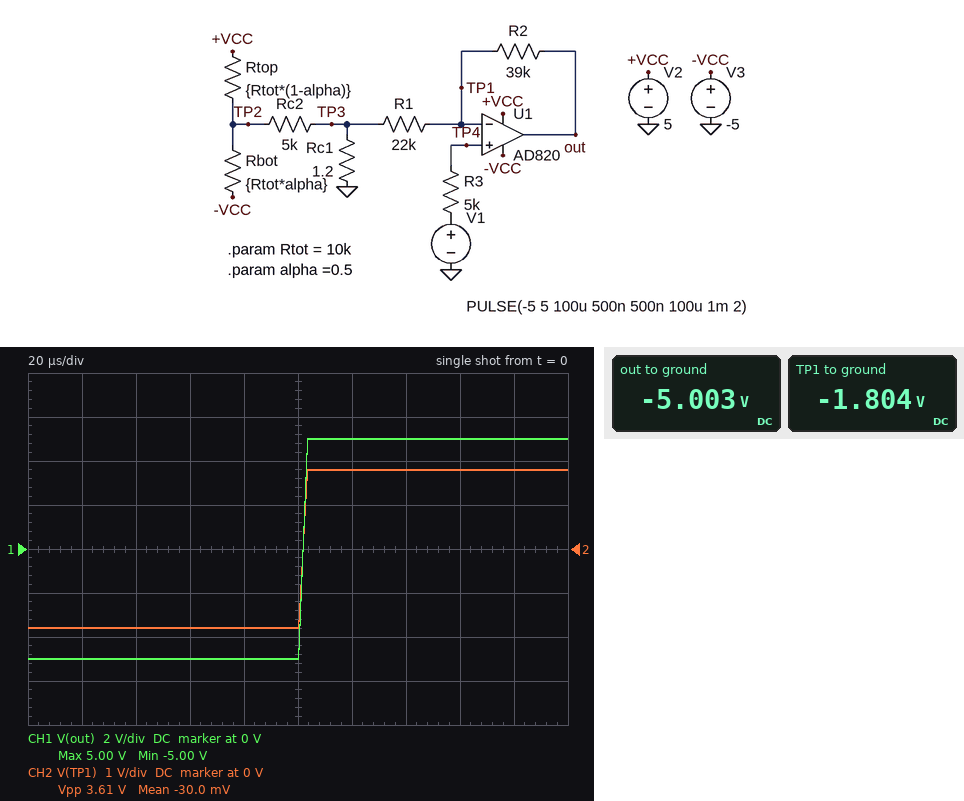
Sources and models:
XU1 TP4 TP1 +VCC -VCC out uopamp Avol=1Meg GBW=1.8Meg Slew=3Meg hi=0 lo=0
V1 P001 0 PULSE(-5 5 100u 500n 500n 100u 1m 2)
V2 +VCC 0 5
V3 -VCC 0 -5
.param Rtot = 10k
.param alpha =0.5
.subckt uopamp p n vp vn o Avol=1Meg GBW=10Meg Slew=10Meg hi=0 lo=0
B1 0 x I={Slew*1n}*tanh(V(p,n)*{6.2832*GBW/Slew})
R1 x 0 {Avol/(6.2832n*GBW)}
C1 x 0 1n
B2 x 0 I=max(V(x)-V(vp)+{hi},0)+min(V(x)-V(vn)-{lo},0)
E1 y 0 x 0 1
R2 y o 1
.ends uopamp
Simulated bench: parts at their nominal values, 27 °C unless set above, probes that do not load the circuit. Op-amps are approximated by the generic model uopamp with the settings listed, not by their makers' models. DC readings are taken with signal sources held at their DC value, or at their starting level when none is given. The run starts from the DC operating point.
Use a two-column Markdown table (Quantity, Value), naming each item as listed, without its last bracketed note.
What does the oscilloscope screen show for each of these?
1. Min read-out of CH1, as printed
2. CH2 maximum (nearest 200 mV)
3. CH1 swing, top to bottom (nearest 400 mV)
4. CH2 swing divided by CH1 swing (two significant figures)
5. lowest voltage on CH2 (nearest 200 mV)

| Quantity | Value |
|---|---|
| Min read-out of CH1, as printed | -5.00 V |
| CH2 maximum | 1.8 V |
| CH1 swing, top to bottom | 10.0 V |
| CH2 swing divided by CH1 swing | 0.36 |
| lowest voltage on CH2 | -1.8 V |
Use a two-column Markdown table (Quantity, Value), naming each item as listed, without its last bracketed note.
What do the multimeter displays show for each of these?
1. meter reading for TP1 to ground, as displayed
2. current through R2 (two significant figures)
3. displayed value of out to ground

| Quantity | Value |
|---|---|
| meter reading for TP1 to ground, as displayed | -1.804 V |
| current through R2 | 82 µA |
| displayed value of out to ground | -5.003 V |
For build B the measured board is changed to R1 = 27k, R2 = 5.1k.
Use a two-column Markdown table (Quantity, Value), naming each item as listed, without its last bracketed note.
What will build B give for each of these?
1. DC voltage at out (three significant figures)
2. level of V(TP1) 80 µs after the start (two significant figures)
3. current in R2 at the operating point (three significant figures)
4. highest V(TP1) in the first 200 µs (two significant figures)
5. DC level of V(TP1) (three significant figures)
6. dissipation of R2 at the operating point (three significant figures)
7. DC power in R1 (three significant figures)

| Quantity | Value |
|---|---|
| DC voltage at out | -5.00 V |
| level of V(TP1) 80 µs after the start | -4.2 V |
| current in R2 at the operating point | 156 µA |
| highest V(TP1) in the first 200 µs | 4.2 V |
| DC level of V(TP1) | -4.21 V |
| dissipation of R2 at the operating point | 124 µW |
| DC power in R1 | 656 µW |
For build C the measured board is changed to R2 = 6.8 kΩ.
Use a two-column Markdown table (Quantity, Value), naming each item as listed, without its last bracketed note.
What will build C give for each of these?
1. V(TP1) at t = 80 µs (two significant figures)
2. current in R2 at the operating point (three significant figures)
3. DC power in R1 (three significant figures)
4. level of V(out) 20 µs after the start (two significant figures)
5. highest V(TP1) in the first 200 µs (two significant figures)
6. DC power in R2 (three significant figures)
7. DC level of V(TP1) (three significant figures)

| Quantity | Value |
|---|---|
| V(TP1) at t = 80 µs | -3.8 V |
| current in R2 at the operating point | 174 µA |
| DC power in R1 | 664 µW |
| level of V(out) 20 µs after the start | -5.0 V |
| highest V(TP1) in the first 200 µs | 3.8 V |
| DC power in R2 | 205 µW |
| DC level of V(TP1) | -3.82 V |
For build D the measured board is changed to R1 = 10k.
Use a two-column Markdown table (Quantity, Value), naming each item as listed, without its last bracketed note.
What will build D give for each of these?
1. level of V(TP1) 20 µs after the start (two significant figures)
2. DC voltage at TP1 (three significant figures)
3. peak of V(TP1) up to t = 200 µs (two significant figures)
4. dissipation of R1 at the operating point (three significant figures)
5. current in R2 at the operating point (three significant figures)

| Quantity | Value |
|---|---|
| level of V(TP1) 20 µs after the start | -1.0 V |
| DC voltage at TP1 | -1.02 V |
| peak of V(TP1) up to t = 200 µs | 1.0 V |
| dissipation of R1 at the operating point | 104 µW |
| current in R2 at the operating point | 102 µA |
